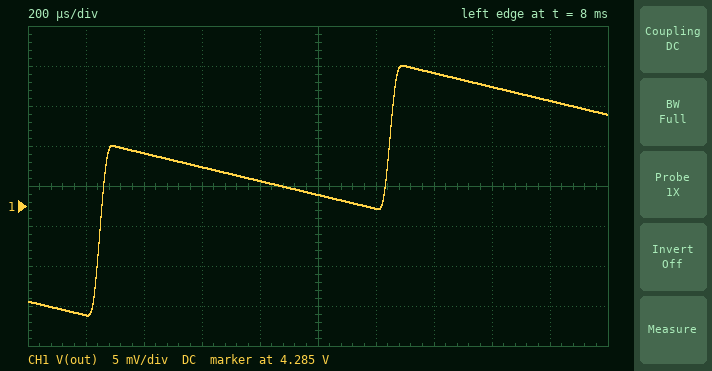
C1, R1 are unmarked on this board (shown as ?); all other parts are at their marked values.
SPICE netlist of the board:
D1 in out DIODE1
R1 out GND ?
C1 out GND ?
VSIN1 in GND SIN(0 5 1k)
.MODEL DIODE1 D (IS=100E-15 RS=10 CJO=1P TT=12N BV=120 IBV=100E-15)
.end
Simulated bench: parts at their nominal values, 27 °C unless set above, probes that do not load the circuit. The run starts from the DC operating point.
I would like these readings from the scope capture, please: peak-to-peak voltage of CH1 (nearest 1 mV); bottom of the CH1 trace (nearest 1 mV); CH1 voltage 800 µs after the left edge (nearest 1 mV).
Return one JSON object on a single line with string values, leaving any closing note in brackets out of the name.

{"peak-to-peak voltage of CH1": "31 mV", "bottom of the CH1 trace": "4.271 V", "CH1 voltage 800 µs after the left edge": "4.288 V"}
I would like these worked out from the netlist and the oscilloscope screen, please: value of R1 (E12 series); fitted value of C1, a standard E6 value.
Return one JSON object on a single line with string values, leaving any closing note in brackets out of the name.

{"value of R1": "33 kΩ", "fitted value of C1, a standard E6 value": "15 µF"}
